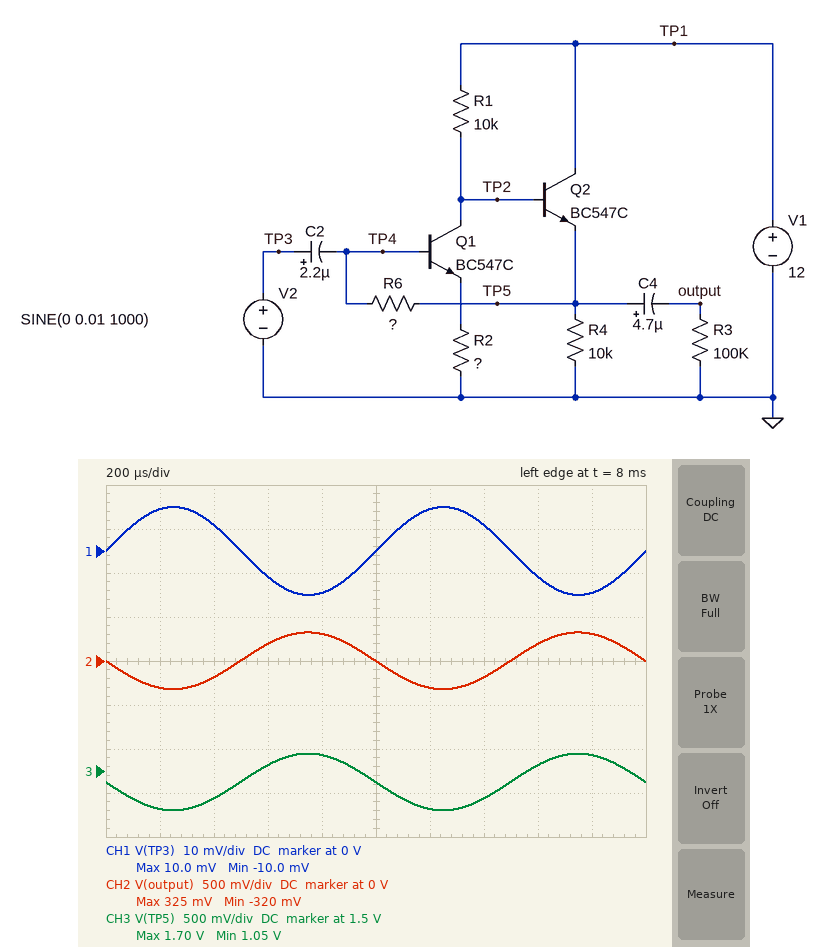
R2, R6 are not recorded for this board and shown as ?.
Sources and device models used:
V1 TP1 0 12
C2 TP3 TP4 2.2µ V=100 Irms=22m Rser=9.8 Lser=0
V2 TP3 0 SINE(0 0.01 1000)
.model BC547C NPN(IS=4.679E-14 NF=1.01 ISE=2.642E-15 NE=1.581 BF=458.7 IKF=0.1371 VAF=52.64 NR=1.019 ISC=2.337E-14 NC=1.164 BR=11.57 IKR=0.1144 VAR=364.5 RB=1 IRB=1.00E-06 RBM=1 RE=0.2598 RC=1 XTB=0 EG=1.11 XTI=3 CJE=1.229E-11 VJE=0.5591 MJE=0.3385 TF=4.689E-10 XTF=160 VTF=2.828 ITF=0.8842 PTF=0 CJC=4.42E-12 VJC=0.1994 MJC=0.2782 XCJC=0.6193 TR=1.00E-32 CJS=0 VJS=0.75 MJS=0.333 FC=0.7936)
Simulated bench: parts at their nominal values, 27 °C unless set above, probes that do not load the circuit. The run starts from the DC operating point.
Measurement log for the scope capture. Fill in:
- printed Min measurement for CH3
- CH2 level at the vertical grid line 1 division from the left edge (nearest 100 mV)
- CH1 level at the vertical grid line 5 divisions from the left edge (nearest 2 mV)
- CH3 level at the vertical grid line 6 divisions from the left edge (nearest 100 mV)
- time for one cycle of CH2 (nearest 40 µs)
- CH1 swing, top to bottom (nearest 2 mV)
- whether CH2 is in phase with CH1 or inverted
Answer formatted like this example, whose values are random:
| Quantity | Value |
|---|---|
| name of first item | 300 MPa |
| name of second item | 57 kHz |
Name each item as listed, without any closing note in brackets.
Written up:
| Quantity | Value |
|---|---|
| printed Min measurement for CH3 | 1.05 V |
| CH2 level at the vertical grid line 1 division from the left edge | -300 mV |
| CH1 level at the vertical grid line 5 divisions from the left edge | 0 V |
| CH3 level at the vertical grid line 6 divisions from the left edge | 1.1 V |
| time for one cycle of CH2 | 1.00 ms |
| CH1 swing, top to bottom | 20 mV |
| whether CH2 is in phase with CH1 or inverted | inverted |
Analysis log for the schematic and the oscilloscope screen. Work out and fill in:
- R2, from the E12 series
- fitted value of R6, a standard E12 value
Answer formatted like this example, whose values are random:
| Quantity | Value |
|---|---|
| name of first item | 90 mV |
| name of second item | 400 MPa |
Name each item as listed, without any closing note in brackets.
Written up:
| Quantity | Value |
|---|---|
| R2, from the E12 series | 270 Ω |
| fitted value of R6, a standard E12 value | 220 kΩ |
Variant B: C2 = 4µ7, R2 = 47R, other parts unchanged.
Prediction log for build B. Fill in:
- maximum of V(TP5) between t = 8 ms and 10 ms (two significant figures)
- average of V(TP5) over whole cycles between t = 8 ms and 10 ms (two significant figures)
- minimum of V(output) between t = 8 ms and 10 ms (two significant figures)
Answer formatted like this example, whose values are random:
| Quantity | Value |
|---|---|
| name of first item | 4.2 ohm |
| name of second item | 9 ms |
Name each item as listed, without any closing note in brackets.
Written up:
| Quantity | Value |
|---|---|
| maximum of V(TP5) between t = 8 ms and 10 ms | 2.4 V |
| average of V(TP5) over whole cycles between t = 8 ms and 10 ms | 1.2 V |
| minimum of V(output) between t = 8 ms and 10 ms | -1.0 V |
